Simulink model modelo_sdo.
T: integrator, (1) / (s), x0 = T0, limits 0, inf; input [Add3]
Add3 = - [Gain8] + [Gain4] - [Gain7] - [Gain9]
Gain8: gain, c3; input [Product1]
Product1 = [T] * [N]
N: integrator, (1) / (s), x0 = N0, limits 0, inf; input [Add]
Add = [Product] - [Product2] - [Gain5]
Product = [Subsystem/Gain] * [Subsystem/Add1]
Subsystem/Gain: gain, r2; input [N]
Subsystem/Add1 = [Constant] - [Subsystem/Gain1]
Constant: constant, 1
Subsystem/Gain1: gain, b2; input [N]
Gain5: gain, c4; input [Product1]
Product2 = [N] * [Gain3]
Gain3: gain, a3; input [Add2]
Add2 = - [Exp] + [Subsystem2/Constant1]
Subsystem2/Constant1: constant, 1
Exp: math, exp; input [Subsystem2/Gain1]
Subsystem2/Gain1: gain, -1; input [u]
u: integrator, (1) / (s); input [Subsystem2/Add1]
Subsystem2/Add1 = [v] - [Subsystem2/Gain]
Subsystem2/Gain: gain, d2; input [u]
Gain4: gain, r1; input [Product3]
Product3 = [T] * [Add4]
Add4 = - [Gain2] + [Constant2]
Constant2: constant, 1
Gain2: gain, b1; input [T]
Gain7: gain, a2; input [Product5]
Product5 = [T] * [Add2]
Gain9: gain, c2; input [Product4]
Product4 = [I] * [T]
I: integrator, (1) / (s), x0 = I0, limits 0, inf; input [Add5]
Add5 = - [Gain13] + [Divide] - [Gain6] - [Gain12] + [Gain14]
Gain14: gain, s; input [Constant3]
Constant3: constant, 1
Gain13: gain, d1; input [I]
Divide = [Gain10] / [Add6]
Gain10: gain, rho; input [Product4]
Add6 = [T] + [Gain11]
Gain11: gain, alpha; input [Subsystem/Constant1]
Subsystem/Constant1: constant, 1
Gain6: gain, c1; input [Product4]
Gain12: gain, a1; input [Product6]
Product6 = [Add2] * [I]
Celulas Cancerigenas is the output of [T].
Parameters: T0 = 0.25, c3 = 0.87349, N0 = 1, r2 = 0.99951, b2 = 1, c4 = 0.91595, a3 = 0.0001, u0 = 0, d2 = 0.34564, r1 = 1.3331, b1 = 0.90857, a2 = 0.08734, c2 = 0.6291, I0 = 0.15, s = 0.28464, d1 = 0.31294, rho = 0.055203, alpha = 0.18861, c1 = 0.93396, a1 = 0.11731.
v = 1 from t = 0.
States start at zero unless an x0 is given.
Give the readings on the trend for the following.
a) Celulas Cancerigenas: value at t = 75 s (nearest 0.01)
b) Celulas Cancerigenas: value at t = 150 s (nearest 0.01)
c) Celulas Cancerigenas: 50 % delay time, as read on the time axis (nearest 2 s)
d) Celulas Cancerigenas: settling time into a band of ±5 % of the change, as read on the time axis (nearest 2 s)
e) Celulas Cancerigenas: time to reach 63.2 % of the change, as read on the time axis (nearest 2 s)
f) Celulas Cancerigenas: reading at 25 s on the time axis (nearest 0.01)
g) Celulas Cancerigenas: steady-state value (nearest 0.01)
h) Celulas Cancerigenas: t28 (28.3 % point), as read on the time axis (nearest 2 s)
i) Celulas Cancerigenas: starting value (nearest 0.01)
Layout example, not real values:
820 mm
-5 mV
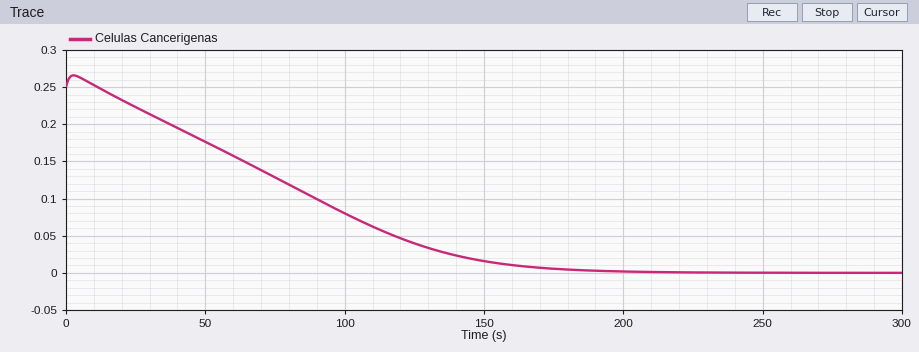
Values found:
0.13
0.02
76 s
156 s
94 s
0.22
0.00
48 s
0.25
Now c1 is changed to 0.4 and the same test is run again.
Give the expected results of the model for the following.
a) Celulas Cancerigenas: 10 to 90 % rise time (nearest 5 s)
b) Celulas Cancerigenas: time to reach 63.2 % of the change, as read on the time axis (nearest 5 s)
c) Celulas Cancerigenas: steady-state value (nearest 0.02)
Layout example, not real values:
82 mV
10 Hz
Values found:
40 s
20 s
0.00
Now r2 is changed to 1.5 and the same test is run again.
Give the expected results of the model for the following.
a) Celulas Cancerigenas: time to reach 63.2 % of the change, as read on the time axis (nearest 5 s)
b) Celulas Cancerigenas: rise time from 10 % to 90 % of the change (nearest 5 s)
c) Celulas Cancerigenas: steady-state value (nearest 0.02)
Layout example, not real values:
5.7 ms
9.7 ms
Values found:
25 s
50 s
0.00
